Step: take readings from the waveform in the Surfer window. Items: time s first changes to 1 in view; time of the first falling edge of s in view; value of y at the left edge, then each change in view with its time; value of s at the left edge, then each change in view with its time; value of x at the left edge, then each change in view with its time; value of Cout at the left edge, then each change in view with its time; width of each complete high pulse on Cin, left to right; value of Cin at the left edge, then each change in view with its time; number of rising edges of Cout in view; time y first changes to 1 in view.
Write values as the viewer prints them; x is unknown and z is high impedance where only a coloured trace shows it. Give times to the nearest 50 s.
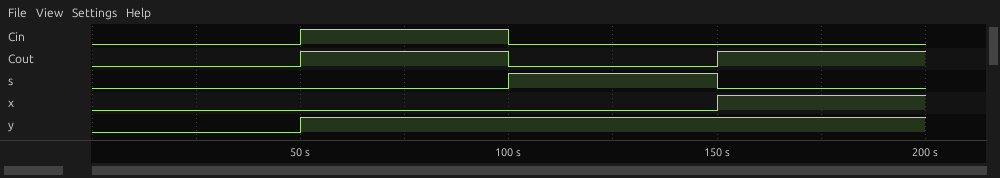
100 s
150 s
0, 1 at 50 s
0, 1 at 100 s, 0 at 150 s
0, 1 at 150 s
0, 1 at 50 s, 0 at 100 s, 1 at 150 s
50 s
0, 1 at 50 s, 0 at 100 s
2
50 s
